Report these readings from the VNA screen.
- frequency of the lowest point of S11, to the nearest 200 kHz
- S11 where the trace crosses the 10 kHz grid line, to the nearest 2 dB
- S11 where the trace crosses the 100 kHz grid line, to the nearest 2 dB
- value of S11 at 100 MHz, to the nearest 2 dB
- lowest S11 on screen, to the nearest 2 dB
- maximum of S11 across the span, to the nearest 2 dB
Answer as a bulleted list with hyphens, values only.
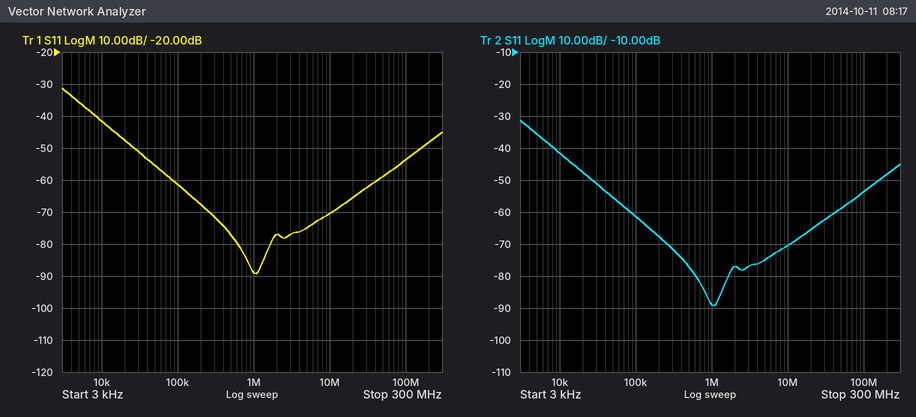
- 1.0 MHz
- -42 dB
- -62 dB
- -54 dB
- -90 dB
- -32 dB
